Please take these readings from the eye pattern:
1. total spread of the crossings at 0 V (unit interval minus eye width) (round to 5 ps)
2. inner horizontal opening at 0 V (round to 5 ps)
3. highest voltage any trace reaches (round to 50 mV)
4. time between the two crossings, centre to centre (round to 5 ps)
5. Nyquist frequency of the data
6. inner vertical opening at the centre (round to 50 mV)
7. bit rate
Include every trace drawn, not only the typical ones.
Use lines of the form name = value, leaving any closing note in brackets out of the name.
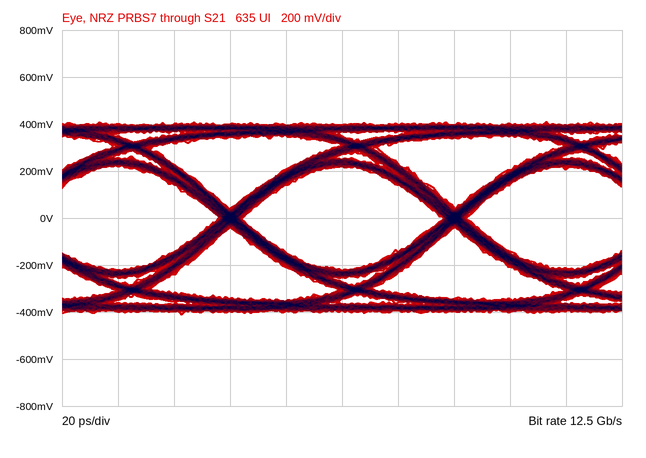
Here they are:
total spread of the crossings at 0 V (unit interval minus eye width) = 10 ps
inner horizontal opening at 0 V = 70 ps
highest voltage any trace reaches = 400 mV
time between the two crossings, centre to centre = 80 ps
Nyquist frequency of the data = 6.25 GHz
inner vertical opening at the centre = 450 mV
bit rate = 12.5 Gb/s
